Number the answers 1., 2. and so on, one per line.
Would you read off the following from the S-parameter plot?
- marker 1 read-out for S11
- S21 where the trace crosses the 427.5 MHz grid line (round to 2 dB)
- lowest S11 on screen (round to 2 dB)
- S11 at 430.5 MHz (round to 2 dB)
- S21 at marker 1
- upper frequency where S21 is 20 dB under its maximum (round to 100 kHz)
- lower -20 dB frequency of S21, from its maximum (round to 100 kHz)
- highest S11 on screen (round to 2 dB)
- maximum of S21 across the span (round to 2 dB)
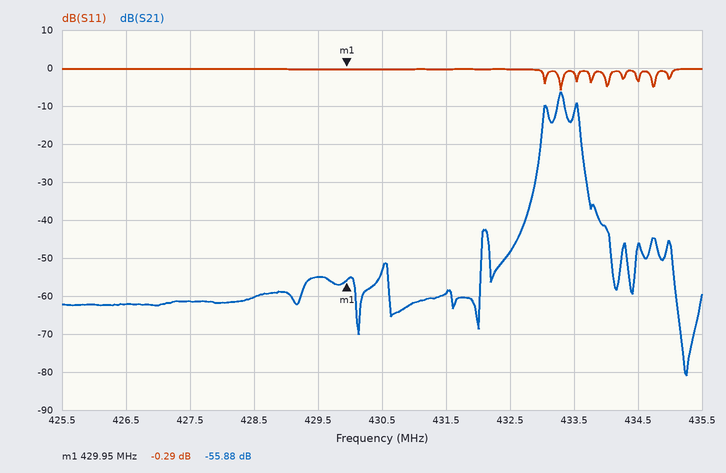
1. -0.29 dB
2. -62 dB
3. -6 dB
4. 0 dB
5. -55.88 dB
6. 433.7 MHz
7. 432.9 MHz
8. 0 dB
9. -6 dB
